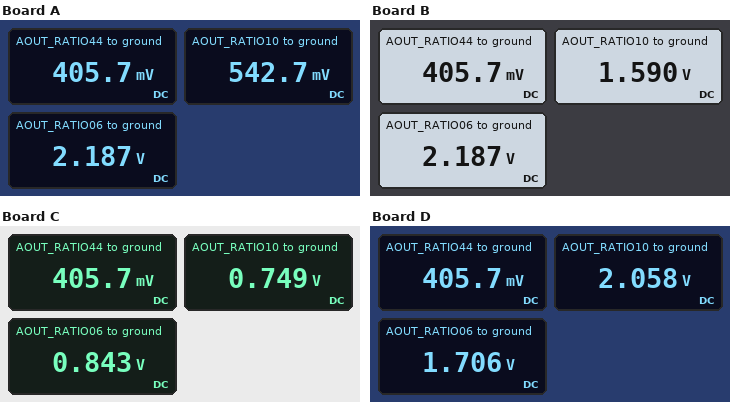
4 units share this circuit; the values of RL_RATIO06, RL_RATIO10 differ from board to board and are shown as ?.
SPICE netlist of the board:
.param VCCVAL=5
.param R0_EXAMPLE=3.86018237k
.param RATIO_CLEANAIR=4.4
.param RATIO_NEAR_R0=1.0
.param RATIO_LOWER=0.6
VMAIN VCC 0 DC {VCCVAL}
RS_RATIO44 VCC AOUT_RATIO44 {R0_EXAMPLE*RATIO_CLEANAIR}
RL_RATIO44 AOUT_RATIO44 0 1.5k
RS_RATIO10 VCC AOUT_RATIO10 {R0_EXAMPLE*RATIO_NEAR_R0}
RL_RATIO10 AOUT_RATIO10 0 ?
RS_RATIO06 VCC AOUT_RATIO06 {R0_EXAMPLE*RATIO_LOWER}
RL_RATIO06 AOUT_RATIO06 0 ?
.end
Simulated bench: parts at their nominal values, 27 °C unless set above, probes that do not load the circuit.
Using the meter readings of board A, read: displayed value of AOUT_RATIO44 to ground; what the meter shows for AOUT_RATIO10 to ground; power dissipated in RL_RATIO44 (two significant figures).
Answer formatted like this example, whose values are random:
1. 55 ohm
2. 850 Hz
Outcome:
1. 405.7 mV
2. 542.7 mV
3. 110 µW
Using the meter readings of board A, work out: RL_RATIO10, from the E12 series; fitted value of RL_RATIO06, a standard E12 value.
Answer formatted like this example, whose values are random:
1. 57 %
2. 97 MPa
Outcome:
1. 470 Ω
2. 1.8 kΩ
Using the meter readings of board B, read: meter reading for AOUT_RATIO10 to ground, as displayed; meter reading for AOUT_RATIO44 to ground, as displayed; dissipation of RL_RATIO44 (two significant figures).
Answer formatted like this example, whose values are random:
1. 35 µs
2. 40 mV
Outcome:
1. 1.590 V
2. 405.7 mV
3. 110 µW
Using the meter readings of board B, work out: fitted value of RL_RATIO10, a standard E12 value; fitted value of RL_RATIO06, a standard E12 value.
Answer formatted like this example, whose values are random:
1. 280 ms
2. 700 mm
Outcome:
1. 1.8 kΩ
2. 1.8 kΩ
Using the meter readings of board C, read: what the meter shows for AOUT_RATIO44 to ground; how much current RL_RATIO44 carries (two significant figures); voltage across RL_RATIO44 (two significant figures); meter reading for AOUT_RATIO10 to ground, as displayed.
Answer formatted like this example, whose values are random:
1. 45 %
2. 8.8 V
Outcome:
1. 405.7 mV
2. 270 µA
3. 410 mV
4. 0.749 V
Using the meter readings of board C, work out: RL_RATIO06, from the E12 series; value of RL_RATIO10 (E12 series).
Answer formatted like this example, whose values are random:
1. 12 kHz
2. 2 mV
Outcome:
1. 470 Ω
2. 680 Ω
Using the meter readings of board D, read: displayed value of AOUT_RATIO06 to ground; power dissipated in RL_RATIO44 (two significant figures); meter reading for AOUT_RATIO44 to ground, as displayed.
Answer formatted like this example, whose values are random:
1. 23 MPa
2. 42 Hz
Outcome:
1. 1.706 V
2. 110 µW
3. 405.7 mV
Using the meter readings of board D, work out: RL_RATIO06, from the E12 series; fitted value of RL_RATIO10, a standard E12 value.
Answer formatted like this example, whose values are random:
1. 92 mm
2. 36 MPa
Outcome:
1. 1.2 kΩ
2. 2.7 kΩ
